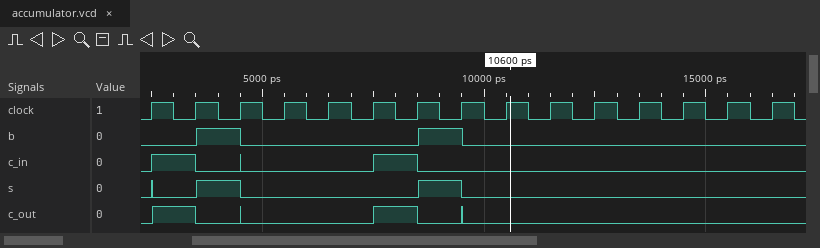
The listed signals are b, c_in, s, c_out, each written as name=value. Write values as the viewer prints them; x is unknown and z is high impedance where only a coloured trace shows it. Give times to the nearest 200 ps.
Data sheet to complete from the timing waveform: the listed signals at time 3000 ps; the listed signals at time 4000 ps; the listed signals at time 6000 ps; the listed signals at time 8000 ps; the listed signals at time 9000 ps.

b=0, c_in=1, s=0, c_out=1
b=1, c_in=0, s=1, c_out=0
b=0, c_in=0, s=0, c_out=0
b=0, c_in=1, s=0, c_out=1
b=1, c_in=0, s=1, c_out=0
